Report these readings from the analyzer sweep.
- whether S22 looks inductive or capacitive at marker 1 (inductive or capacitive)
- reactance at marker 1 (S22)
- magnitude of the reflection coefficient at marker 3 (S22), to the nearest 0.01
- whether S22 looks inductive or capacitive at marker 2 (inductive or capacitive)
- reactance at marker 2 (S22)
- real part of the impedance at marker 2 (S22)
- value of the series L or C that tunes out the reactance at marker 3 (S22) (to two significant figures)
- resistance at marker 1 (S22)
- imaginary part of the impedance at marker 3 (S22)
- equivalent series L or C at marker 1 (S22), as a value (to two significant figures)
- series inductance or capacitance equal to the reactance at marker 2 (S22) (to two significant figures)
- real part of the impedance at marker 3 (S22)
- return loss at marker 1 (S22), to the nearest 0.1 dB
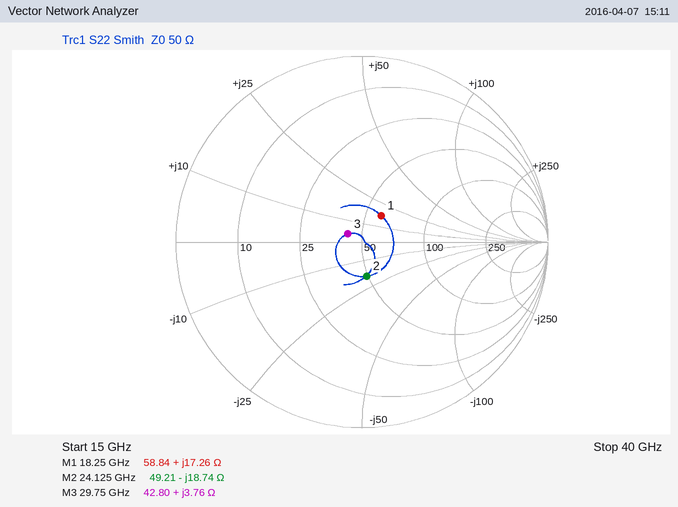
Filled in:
inductive
+17.26 Ω
0.09
capacitive
-18.74 Ω
49.21 Ω
1.4 pF
58.84 Ω
+3.76 Ω
150 pH
350 fF
42.80 Ω
15.1 dB
